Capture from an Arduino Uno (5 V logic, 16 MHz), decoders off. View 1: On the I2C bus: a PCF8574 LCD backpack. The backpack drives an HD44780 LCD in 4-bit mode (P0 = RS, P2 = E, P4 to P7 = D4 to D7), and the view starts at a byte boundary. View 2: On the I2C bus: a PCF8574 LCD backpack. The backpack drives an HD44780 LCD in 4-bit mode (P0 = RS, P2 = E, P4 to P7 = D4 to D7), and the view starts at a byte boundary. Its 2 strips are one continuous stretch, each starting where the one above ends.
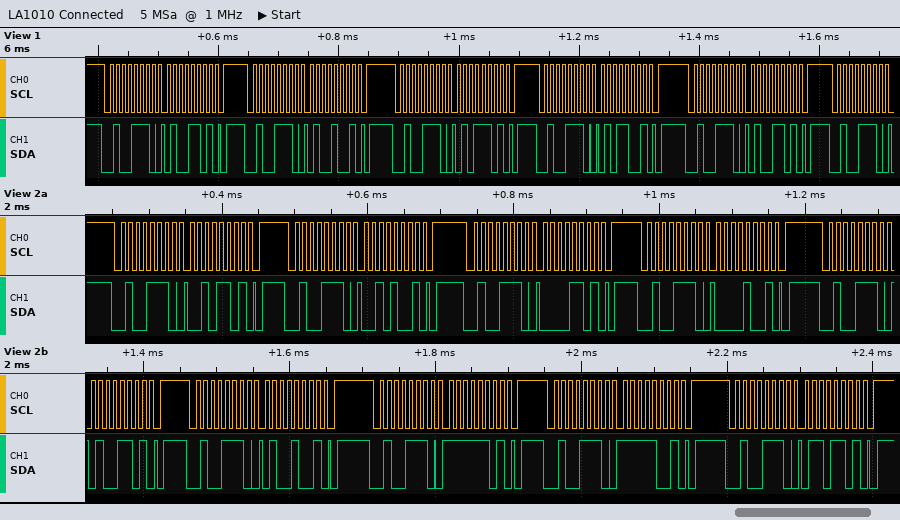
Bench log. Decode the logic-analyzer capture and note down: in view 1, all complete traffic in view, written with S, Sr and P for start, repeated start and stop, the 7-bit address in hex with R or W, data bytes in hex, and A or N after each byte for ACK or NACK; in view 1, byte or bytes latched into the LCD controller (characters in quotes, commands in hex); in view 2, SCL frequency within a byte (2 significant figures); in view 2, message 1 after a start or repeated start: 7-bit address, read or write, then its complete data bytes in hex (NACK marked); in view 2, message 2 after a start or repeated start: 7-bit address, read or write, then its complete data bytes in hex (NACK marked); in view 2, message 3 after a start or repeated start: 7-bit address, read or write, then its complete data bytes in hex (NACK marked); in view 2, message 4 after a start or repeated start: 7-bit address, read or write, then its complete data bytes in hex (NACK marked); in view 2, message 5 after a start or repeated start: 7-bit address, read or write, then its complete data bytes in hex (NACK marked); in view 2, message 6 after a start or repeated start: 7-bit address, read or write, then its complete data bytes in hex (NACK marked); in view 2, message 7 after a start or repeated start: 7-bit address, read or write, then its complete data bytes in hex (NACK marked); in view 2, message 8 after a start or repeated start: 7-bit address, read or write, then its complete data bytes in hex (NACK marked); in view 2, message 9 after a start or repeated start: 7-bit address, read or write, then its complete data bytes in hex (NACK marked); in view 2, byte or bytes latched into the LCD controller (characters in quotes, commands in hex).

S 27W A 4D A P S 27W A 49 A P S 27W A 5D A P S 27W A 59 A P S 27W A 4D A P S 27W A
'E'
100 kHz
0x27 write: 2D
0x27 write: 29
0x27 write: 0D
0x27 write: 09
0x27 write: 4D
0x27 write: 49
0x27 write: FD
0x27 write: F9
0x27 write: 6D
' ' 'O'
